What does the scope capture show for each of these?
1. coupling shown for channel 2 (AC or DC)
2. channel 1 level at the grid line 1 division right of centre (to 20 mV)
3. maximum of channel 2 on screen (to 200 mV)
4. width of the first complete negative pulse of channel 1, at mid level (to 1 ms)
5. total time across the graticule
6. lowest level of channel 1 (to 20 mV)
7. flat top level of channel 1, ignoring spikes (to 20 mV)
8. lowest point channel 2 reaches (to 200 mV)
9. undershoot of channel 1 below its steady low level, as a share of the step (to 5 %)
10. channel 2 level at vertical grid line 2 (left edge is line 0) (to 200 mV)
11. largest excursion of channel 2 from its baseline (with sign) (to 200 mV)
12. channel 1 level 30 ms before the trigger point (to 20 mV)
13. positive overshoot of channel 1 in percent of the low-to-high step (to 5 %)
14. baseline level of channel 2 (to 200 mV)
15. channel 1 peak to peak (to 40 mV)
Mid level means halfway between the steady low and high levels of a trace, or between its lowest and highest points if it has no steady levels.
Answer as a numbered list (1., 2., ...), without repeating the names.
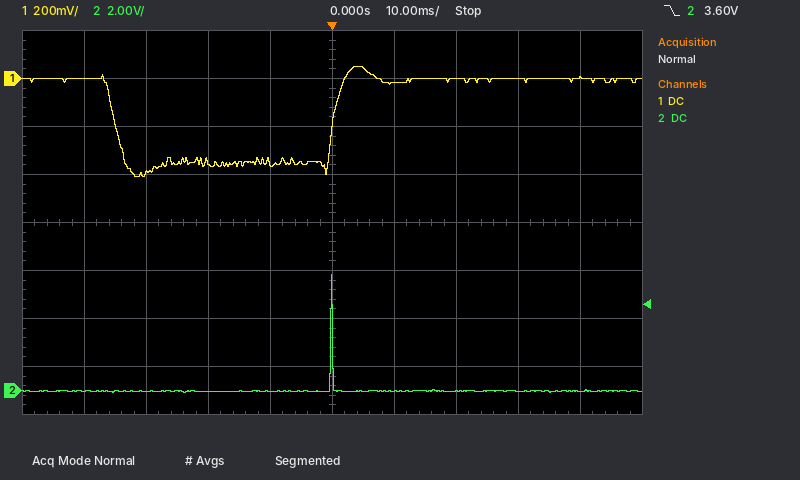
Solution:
1. DC
2. -20 mV
3. 4.8 V
4. 35 ms
5. 100 ms
6. -400 mV
7. 0 mV
8. 0.0 V
9. 15 %
10. 0.0 V
11. +4.8 V
12. -400 mV
13. 15 %
14. 0.0 V
15. 440 mV
